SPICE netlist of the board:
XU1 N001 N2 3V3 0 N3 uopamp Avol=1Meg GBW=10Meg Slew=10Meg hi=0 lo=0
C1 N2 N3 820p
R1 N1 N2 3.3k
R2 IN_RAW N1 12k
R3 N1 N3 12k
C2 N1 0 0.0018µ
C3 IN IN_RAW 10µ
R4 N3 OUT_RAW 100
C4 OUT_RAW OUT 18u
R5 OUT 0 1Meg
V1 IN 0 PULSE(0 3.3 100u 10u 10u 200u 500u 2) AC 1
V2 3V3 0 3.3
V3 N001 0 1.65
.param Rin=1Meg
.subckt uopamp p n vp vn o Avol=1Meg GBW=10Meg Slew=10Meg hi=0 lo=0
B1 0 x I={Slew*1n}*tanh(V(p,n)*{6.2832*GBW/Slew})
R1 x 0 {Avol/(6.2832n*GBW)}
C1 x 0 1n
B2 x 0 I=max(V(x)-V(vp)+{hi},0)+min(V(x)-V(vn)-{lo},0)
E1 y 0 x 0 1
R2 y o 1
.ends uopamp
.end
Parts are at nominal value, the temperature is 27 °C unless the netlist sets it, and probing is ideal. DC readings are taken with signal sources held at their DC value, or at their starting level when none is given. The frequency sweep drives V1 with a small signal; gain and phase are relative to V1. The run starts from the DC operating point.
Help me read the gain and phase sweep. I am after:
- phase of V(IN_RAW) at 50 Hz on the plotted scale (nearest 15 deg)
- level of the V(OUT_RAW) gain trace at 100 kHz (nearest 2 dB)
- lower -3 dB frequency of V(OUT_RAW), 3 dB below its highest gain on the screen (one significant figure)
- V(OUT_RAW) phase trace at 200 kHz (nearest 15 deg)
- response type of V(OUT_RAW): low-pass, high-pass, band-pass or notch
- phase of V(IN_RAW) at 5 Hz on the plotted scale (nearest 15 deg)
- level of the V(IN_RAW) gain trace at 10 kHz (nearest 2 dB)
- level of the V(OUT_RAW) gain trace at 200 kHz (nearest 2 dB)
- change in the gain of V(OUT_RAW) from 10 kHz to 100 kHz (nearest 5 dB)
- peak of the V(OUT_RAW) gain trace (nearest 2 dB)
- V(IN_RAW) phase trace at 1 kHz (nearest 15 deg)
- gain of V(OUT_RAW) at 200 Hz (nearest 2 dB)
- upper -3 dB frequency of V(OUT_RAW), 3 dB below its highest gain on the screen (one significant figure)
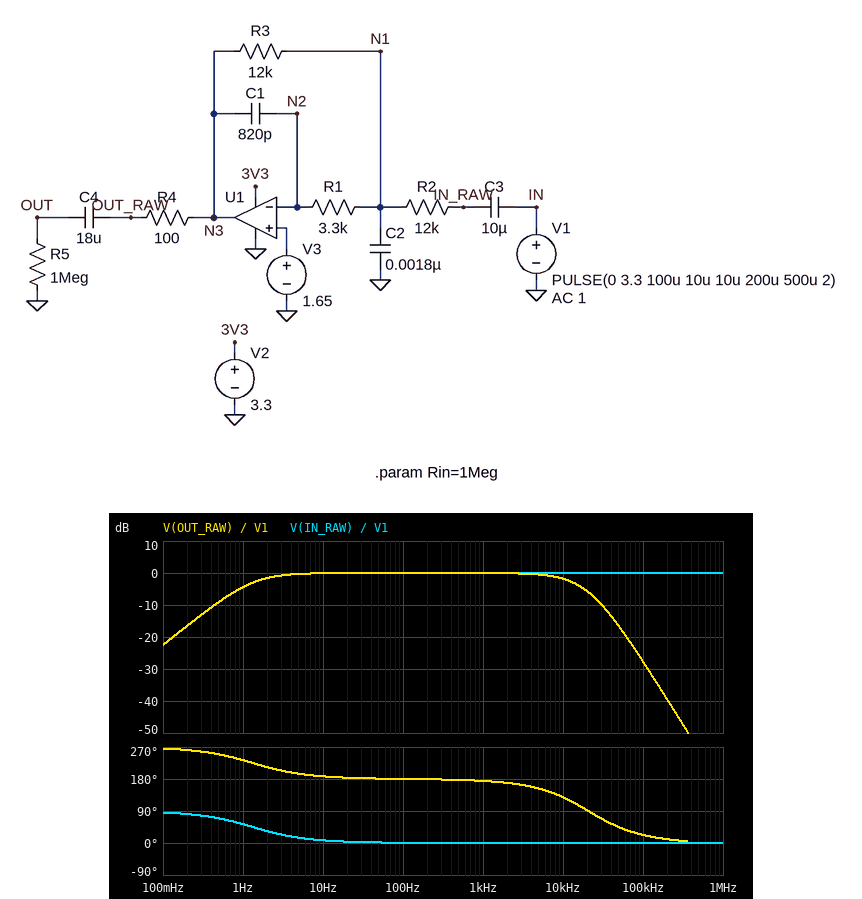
0 deg
-28 dB
1 Hz
15 deg
band-pass
15 deg
0 dB
-40 dB
-25 dB
0 dB
0 deg
0 dB
10 kHz
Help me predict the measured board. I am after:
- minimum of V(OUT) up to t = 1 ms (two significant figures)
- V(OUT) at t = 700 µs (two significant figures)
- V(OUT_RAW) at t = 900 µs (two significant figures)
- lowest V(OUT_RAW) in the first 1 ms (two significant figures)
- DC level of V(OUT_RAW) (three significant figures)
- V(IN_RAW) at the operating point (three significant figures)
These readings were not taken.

-1.7 V
-1.7 V
1.7 V
-9.7 mV
1.65 V
1.65 V
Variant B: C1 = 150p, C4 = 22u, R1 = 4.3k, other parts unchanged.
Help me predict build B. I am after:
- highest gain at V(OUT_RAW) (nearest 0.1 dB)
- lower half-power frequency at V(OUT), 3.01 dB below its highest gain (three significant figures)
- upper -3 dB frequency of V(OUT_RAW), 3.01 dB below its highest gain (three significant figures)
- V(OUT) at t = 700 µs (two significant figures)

2.5 dB
3.78 Hz
50.0 kHz
-1.7 V
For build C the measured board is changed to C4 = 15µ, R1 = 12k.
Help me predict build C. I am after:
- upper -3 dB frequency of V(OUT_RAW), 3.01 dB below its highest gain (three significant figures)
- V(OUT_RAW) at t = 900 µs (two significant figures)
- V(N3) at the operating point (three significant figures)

6.90 kHz
1.6 V
1.65 V
